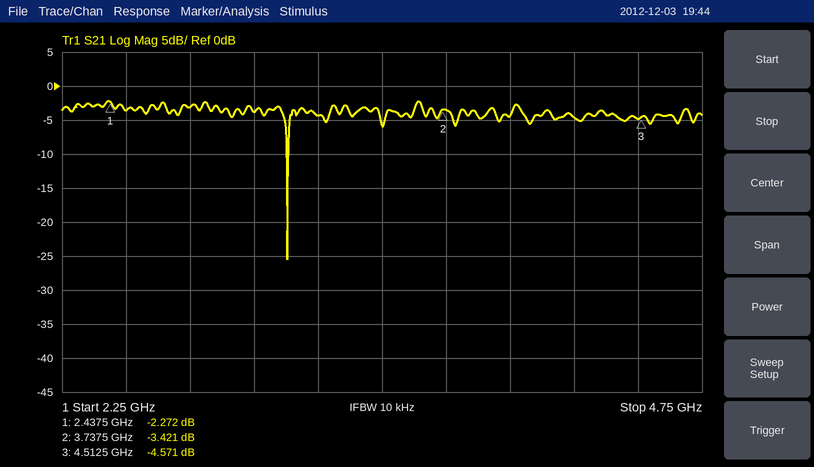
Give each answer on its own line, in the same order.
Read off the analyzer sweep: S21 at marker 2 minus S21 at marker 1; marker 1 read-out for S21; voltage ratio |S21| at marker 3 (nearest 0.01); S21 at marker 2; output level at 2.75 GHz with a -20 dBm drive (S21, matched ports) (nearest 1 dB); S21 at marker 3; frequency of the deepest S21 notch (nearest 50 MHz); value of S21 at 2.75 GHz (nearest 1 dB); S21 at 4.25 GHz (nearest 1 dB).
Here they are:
-1.149 dB
-2.272 dB
0.59
-3.421 dB
-23 dBm
-4.571 dB
3.15 GHz
-3 dB
-5 dB
